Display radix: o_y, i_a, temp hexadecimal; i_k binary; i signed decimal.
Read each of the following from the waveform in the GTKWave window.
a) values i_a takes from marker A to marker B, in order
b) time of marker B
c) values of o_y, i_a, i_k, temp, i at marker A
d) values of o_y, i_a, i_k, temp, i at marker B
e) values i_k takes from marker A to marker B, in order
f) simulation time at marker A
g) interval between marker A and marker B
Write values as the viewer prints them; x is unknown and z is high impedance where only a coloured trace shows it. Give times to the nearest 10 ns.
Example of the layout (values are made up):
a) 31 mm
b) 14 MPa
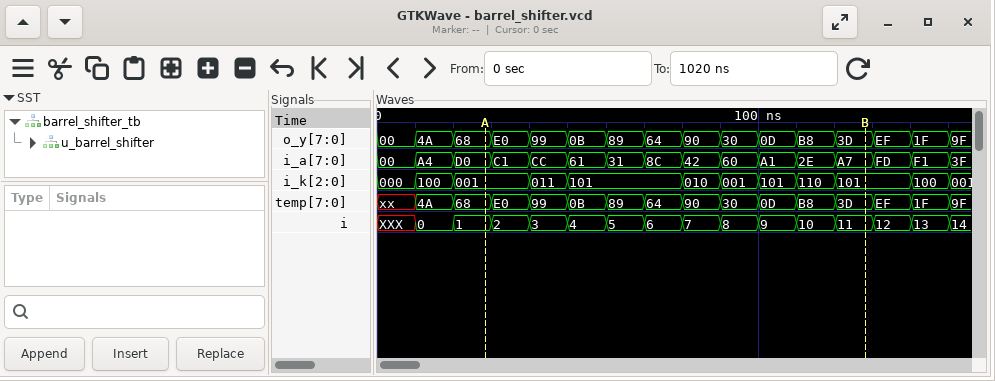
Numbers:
a) D0, C1, CC, 61, 31, 8C, 42, 60, A1, 2E, A7
b) 130 ns
c) o_y=68, i_a=D0, i_k=001, temp=68, i=1
d) o_y=3D, i_a=A7, i_k=101, temp=3D, i=11
e) 001, 011, 101, 010, 001, 101, 110, 101
f) 30 ns
g) 100 ns
